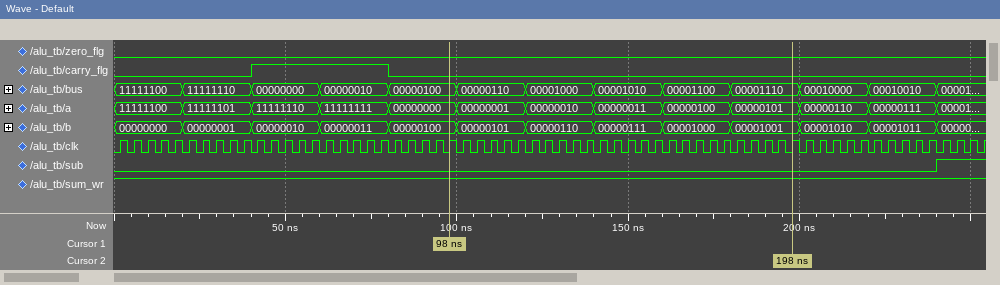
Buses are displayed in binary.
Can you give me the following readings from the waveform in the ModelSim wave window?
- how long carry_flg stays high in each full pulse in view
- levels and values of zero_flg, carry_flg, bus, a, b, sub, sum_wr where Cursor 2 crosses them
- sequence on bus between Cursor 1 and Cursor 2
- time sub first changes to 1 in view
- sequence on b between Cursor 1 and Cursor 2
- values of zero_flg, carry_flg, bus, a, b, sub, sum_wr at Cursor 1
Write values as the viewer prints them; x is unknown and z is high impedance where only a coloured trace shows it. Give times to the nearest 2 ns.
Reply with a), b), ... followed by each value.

a) 40 ns
b) zero_flg=0, carry_flg=0, bus=00001110, a=00000101, b=00001001, sub=0, sum_wr=1
c) 00000100, 00000110, 00001000, 00001010, 00001100, 00001110
d) 240 ns
e) 00000100, 00000101, 00000110, 00000111, 00001000, 00001001
f) zero_flg=0, carry_flg=0, bus=00000100, a=00000000, b=00000100, sub=0, sum_wr=1
